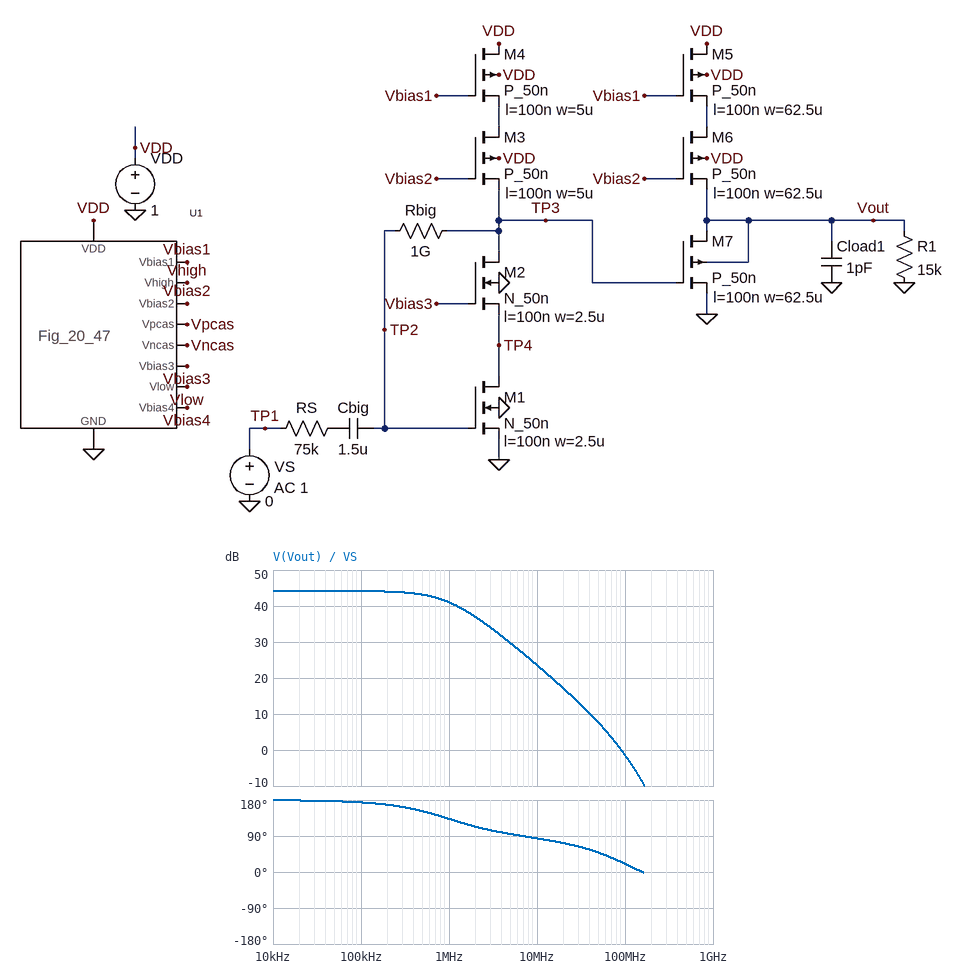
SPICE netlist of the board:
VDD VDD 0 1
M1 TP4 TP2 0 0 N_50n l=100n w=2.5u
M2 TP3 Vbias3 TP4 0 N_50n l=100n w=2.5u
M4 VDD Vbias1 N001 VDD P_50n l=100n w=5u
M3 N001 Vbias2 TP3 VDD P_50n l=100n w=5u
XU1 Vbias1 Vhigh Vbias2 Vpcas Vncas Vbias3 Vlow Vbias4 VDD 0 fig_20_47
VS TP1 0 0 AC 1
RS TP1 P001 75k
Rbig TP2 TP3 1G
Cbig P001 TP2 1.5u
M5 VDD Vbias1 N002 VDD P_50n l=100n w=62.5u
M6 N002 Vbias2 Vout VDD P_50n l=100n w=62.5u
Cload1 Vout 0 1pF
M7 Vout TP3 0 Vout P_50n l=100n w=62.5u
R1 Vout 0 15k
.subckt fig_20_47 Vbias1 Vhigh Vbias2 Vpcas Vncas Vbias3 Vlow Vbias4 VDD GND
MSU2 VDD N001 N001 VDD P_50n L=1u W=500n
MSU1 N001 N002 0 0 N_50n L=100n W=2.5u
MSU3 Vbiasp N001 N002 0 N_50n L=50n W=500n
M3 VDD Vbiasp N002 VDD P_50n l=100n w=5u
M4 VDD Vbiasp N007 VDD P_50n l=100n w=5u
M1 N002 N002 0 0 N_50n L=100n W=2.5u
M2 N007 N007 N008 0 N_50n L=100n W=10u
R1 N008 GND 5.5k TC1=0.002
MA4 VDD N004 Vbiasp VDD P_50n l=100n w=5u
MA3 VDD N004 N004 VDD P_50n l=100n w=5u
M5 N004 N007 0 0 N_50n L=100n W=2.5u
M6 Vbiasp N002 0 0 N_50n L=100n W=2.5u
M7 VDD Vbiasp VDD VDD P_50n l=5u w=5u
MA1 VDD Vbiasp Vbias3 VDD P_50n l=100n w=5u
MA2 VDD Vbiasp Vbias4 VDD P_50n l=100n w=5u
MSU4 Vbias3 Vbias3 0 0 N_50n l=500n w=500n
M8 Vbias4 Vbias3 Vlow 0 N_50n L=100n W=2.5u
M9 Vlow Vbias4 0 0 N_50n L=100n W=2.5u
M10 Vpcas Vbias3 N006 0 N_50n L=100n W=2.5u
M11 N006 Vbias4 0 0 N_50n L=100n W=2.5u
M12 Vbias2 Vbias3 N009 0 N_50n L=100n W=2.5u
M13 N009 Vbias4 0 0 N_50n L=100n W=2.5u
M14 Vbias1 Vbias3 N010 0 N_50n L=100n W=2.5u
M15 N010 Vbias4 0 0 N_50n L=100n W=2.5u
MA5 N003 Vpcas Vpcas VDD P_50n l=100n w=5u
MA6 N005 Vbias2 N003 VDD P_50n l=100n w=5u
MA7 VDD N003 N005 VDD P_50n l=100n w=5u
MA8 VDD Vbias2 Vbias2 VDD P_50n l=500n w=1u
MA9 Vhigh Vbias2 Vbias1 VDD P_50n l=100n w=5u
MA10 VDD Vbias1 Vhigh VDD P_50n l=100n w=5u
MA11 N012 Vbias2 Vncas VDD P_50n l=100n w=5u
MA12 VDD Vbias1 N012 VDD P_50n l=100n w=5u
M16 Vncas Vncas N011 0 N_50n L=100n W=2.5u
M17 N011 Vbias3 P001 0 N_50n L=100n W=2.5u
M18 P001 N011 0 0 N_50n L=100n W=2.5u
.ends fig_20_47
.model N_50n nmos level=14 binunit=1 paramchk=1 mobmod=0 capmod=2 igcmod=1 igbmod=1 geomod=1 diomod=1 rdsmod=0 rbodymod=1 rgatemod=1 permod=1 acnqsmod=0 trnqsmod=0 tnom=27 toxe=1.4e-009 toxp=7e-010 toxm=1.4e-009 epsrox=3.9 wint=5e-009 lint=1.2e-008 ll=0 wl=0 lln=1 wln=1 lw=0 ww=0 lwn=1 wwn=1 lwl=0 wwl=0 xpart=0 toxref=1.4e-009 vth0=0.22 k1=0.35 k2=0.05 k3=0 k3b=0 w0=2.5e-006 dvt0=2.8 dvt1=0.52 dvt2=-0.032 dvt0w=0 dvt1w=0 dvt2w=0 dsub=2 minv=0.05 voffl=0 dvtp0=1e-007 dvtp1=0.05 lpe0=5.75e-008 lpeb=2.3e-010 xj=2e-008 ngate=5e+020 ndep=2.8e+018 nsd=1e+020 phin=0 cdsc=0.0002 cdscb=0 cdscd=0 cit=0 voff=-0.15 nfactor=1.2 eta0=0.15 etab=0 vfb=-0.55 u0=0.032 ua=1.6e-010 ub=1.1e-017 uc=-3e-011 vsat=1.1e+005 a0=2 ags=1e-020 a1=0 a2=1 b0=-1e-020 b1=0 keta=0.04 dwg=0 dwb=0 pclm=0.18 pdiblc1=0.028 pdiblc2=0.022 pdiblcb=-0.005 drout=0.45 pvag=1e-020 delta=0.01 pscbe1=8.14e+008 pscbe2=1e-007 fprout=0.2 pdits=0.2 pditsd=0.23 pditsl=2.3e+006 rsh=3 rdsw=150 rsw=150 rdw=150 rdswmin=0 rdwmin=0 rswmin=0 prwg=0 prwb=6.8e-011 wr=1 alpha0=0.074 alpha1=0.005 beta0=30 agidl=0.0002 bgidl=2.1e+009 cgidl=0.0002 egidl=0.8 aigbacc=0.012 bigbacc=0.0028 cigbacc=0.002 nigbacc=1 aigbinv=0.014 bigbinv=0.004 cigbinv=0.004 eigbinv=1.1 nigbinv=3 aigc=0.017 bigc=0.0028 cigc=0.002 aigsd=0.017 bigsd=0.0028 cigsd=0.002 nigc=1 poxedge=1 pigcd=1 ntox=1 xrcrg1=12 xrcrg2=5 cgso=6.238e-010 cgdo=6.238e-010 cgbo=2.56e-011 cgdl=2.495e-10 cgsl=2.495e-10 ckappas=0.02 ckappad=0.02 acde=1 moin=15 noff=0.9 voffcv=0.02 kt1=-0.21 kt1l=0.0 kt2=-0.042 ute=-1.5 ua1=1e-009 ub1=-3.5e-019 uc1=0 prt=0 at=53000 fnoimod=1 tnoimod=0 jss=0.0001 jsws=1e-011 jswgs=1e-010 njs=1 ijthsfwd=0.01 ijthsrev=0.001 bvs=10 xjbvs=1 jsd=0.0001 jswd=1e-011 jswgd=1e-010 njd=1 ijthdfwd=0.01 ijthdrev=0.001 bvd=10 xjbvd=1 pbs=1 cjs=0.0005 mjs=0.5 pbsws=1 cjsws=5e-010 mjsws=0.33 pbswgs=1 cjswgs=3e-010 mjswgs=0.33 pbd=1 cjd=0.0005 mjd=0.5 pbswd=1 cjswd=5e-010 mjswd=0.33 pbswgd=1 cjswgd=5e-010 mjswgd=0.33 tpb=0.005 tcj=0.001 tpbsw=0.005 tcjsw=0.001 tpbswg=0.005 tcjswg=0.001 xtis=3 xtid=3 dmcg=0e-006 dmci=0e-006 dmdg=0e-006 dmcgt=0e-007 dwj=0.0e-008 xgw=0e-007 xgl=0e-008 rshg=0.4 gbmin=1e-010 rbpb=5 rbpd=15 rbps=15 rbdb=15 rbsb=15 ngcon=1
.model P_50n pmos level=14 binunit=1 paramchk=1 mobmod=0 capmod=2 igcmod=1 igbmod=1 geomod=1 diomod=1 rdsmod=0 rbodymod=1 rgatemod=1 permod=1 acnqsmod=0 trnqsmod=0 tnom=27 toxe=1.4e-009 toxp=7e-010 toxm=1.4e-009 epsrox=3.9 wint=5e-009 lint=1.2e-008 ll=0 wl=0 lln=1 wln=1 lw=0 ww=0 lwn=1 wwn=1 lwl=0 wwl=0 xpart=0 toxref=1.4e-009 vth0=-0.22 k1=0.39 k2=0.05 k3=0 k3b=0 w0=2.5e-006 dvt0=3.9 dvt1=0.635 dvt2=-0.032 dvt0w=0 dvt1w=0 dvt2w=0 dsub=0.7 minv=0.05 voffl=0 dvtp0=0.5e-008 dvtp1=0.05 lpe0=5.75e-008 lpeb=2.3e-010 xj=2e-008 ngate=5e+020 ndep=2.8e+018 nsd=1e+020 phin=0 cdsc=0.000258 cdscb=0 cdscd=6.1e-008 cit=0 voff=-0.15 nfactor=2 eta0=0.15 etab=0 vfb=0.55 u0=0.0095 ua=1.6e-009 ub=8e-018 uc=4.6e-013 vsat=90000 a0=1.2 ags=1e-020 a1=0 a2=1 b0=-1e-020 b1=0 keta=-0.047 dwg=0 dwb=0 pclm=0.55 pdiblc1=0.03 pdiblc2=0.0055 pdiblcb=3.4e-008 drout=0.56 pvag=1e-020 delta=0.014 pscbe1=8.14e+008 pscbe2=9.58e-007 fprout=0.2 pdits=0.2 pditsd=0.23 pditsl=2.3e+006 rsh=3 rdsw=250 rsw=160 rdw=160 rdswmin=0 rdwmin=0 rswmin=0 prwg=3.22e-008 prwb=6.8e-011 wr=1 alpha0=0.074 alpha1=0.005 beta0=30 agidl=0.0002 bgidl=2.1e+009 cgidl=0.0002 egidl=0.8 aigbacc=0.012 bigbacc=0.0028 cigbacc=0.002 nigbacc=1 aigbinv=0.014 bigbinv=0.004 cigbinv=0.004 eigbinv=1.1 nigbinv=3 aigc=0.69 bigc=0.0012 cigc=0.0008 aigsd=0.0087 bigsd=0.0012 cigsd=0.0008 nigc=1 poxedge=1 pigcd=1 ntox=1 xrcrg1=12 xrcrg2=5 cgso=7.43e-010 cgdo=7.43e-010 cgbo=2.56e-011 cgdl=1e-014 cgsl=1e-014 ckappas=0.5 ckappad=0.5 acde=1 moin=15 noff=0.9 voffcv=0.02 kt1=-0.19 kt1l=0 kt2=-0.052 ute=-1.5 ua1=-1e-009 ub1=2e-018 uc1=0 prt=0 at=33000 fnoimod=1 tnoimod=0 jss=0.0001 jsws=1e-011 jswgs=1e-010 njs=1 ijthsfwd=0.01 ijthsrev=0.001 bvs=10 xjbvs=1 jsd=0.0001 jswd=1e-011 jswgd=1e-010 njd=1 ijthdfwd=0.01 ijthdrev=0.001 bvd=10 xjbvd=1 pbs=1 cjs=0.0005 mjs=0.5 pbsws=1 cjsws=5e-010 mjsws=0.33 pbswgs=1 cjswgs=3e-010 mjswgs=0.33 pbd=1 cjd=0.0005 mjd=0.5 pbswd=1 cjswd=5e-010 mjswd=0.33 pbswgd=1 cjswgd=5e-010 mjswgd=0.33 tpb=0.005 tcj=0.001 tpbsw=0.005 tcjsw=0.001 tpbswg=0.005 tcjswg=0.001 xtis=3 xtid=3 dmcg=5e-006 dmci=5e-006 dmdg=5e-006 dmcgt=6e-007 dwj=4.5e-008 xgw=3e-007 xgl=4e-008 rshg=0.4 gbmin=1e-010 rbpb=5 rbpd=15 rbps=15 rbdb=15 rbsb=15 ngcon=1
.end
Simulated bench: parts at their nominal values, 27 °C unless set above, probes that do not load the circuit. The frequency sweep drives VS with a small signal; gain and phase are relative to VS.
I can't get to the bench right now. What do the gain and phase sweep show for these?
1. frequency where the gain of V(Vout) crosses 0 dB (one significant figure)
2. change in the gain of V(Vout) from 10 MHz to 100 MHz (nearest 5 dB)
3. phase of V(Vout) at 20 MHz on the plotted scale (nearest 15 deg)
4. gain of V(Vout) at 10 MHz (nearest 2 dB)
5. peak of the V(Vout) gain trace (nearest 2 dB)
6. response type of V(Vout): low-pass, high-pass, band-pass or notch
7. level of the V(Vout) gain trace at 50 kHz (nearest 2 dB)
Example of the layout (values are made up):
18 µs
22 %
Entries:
90 MHz
-25 dB
75 deg
24 dB
44 dB
low-pass
44 dB
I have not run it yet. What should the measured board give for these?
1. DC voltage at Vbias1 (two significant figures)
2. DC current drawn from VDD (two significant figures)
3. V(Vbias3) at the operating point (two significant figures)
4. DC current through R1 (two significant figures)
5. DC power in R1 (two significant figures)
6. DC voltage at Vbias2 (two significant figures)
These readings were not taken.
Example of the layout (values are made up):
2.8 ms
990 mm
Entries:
640 mV
240 µA
540 mV
57 µA
49 µW
370 mV
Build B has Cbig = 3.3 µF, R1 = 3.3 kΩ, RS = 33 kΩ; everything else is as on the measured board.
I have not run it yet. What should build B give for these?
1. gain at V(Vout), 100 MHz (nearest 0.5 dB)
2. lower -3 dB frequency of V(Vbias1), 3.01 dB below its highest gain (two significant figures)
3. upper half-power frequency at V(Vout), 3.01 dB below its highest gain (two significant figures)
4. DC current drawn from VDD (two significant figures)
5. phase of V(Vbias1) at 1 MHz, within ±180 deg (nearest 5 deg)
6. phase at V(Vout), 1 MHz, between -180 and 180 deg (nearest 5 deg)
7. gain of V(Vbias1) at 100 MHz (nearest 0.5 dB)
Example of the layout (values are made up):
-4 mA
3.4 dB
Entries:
-24.5 dB
6.0 MHz
25 MHz
250 µA
25 deg
-155 deg
-52.5 dB
